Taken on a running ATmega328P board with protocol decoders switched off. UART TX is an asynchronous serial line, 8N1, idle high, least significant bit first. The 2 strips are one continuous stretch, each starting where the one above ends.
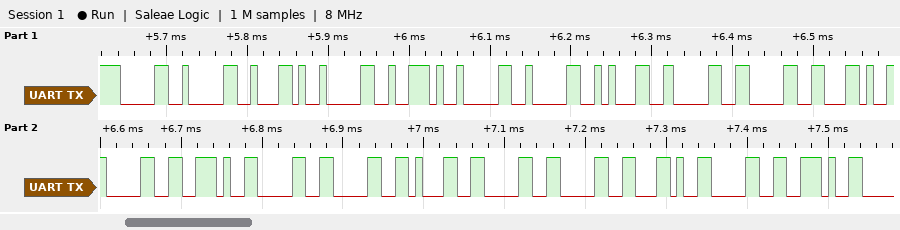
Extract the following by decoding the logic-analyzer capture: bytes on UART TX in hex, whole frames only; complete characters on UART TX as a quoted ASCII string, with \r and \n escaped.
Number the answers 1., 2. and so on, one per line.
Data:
1. 0x30 0x30 0x2C 0x30 0x2E 0x30 0x30 0x31 0x30 0x30 0x2C 0x30 0x2E 0x30 0x30 0x31 0x30 0x30 0x2C 0x30 0x2E
2. "00,0.00100,0.00100,0."
